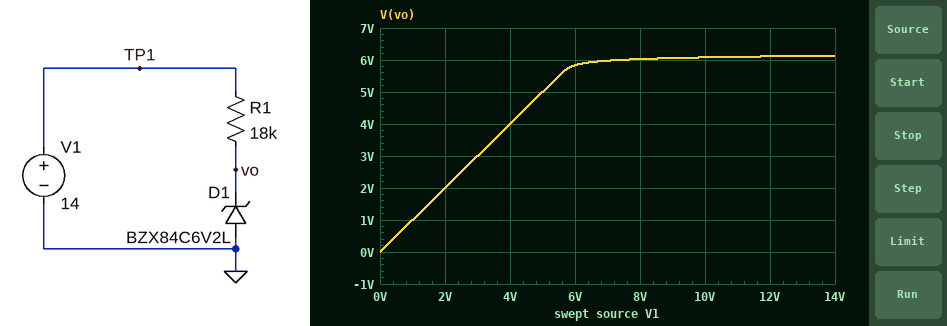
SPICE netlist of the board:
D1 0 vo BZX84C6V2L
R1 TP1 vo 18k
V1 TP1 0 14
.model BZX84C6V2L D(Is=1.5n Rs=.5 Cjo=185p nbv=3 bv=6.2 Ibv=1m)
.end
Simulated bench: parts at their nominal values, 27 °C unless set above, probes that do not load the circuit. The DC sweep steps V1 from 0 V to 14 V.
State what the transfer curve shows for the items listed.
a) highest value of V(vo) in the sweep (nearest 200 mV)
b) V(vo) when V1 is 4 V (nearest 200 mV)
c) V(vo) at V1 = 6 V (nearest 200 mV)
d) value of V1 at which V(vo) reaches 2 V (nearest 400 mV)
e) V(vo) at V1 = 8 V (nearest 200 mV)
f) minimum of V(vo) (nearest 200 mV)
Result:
6.2 V
4.0 V
5.8 V
2.0 V
6.0 V
0 V
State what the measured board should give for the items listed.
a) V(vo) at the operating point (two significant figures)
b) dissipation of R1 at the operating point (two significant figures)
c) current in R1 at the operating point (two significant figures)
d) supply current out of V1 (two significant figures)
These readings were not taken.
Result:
6.1 V
3.4 mW
440 µA
440 µA
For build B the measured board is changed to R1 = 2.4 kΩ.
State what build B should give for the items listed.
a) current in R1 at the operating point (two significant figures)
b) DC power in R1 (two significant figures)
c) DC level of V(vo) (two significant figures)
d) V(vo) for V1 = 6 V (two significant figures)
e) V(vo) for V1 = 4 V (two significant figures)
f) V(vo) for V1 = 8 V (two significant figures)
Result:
3.2 mA
25 mW
6.3 V
5.9 V
4.0 V
6.2 V
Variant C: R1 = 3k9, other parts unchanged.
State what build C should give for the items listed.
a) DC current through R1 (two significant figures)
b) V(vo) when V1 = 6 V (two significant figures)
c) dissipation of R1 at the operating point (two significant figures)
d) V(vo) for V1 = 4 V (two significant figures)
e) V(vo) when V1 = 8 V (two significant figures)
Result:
2.0 mA
5.9 V
15 mW
4.0 V
6.1 V
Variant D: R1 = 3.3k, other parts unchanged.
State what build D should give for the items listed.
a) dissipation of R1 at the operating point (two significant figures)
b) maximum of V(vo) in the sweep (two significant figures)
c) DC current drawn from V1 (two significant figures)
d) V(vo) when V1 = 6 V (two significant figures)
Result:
18 mW
6.3 V
2.3 mA
5.9 V
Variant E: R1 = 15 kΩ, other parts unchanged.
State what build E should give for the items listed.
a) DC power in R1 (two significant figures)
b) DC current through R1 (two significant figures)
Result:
4.1 mW
520 µA
